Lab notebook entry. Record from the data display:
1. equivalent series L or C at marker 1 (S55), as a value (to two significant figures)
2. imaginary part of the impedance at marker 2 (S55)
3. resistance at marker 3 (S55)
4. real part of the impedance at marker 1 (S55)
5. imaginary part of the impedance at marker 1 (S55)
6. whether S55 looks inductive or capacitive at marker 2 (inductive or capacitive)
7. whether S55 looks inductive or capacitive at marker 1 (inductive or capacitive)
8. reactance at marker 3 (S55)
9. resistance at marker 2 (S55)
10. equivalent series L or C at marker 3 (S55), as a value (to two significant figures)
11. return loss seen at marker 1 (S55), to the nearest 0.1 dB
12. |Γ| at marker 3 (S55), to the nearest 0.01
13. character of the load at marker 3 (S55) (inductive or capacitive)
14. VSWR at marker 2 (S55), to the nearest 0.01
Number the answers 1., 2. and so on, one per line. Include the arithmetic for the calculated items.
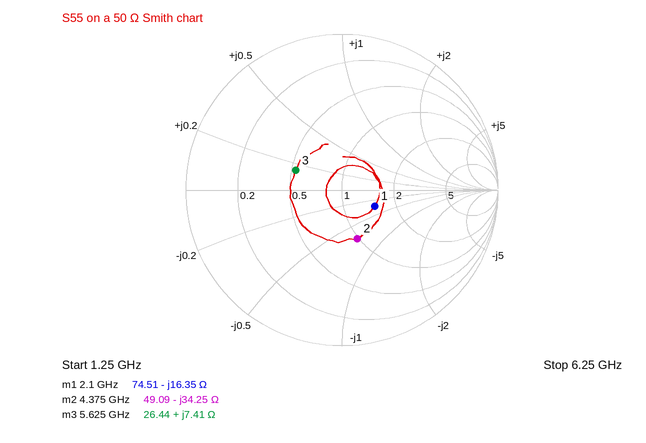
1. C = 1/(2π × 2.1 GHz × 16.35 Ω) ≈ 4.6 pF
2. -34.25 Ω
3. 26.44 Ω
4. 74.51 Ω
5. -16.35 Ω
6. capacitive
7. capacitive
8. +7.41 Ω
9. 49.09 Ω
10. L = 7.41 Ω/(2π × 5.625 GHz) ≈ 210 pH
11. 12.6 dB
12. 0.32
13. inductive
14. 1.97
